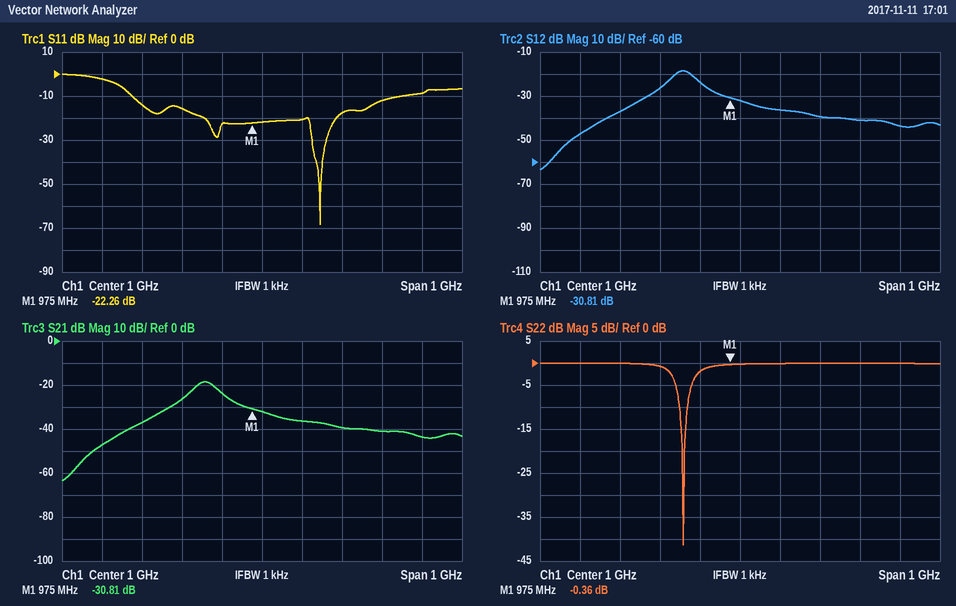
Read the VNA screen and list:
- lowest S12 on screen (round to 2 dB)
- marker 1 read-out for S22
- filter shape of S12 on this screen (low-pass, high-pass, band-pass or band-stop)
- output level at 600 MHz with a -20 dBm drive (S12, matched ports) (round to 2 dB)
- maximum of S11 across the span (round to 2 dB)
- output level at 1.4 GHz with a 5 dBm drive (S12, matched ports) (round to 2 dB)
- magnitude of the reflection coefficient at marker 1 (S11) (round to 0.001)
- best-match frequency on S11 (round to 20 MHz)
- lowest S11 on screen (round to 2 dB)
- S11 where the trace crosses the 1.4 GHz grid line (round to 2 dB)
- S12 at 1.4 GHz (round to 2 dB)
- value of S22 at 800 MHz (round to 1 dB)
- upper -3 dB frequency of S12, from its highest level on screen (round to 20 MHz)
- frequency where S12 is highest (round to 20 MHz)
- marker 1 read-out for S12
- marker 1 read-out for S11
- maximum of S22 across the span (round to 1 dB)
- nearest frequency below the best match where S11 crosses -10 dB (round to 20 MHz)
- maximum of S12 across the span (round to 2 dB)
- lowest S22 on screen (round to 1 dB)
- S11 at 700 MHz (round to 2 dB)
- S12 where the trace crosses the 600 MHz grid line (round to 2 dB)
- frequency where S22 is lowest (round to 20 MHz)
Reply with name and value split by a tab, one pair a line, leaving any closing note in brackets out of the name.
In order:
lowest S12 on screen	-64 dB
marker 1 read-out for S22	-0.36 dB
filter shape of S12 on this screen	band-pass
output level at 600 MHz with a -20 dBm drive (S12, matched ports)	-68 dBm
maximum of S11 across the span	0 dB
output level at 1.4 GHz with a 5 dBm drive (S12, matched ports)	-38 dBm
magnitude of the reflection coefficient at marker 1 (S11)	0.077
best-match frequency on S11	1.14 GHz
lowest S11 on screen	-68 dB
S11 where the trace crosses the 1.4 GHz grid line	-8 dB
S12 at 1.4 GHz	-44 dB
value of S22 at 800 MHz	-1 dB
upper -3 dB frequency of S12, from its highest level on screen	880 MHz
frequency where S12 is highest	860 MHz
marker 1 read-out for S12	-30.81 dB
marker 1 read-out for S11	-22.26 dB
maximum of S22 across the span	0 dB
nearest frequency below the best match where S11 crosses -10 dB	680 MHz
maximum of S12 across the span	-18 dB
lowest S22 on screen	-41 dB
S11 at 700 MHz	-14 dB
S12 where the trace crosses the 600 MHz grid line	-48 dB
frequency where S22 is lowest	860 MHz
